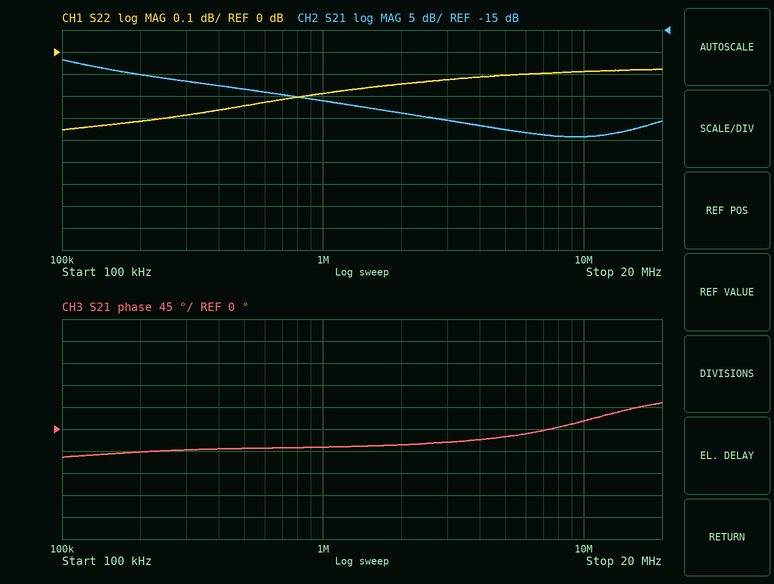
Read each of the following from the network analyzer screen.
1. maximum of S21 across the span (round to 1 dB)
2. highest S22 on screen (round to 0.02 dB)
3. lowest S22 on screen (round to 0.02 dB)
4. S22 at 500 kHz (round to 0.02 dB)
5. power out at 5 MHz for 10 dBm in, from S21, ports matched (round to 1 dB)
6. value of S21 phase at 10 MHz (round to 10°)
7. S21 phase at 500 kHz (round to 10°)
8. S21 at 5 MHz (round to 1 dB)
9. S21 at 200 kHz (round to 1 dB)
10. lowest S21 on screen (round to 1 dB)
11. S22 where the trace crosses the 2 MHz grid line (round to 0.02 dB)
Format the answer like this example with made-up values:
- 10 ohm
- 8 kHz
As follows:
- -22 dB
- -0.08 dB
- -0.36 dB
- -0.24 dB
- -28 dBm
- 20°
- -40°
- -38 dB
- -25 dB
- -39 dB
- -0.14 dB
